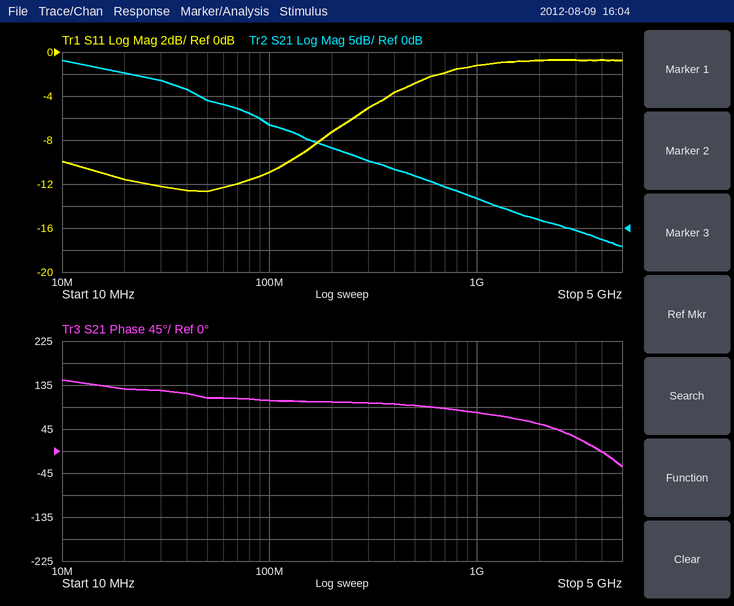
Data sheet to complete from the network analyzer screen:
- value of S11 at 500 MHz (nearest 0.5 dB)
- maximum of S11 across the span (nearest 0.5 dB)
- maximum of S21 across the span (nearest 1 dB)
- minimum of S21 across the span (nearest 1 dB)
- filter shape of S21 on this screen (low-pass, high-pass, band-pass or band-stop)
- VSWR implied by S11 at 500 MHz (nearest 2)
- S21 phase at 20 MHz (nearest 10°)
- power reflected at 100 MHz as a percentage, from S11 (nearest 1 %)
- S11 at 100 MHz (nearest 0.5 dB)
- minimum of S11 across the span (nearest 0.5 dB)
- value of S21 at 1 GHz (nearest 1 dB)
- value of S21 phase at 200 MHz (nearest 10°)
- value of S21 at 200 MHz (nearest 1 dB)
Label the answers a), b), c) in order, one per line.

a) -3.0 dB
b) -0.5 dB
c) 38 dB
d) -4 dB
e) low-pass
f) 6
g) 130°
h) 8 %
i) -11.0 dB
j) -12.5 dB
k) 7 dB
l) 100°
m) 18 dB
